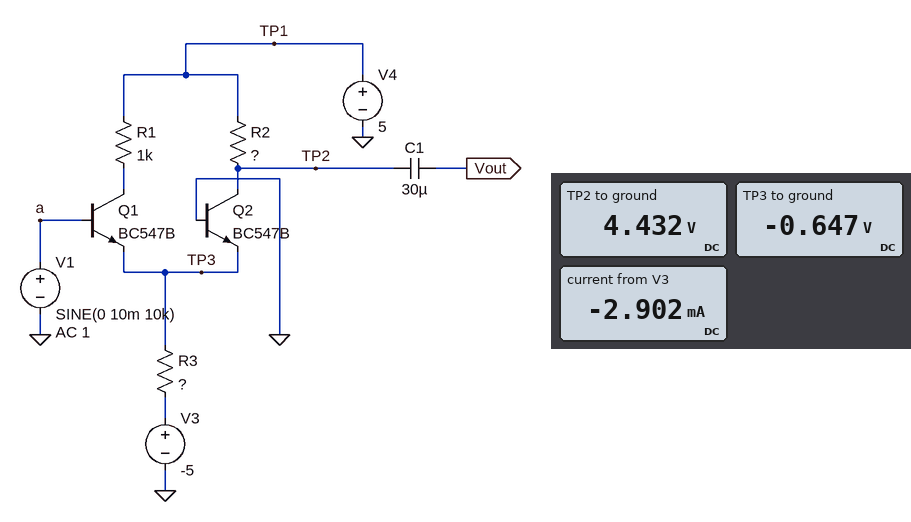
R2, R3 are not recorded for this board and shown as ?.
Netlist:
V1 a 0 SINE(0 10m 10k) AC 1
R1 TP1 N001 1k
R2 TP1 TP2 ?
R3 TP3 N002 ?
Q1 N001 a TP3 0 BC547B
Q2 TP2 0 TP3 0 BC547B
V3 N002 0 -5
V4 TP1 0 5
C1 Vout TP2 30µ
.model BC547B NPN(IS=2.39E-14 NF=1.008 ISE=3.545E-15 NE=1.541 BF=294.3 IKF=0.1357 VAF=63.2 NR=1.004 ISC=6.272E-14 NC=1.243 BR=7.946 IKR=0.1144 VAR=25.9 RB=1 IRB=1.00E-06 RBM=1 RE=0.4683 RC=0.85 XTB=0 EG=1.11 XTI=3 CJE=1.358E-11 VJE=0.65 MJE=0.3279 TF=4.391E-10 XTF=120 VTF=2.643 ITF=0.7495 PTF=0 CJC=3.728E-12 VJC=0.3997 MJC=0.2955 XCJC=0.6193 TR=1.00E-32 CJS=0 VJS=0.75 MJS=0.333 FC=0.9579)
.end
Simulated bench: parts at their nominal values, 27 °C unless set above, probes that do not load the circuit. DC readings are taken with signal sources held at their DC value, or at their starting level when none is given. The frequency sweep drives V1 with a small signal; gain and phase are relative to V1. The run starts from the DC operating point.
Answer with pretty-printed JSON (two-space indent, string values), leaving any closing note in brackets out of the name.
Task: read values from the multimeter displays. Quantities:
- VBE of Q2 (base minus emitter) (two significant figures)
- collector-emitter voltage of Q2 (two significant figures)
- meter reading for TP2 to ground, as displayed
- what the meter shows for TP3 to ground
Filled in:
{
  "VBE of Q2 (base minus emitter)": "650 mV",
  "collector-emitter voltage of Q2": "5.1 V",
  "meter reading for TP2 to ground, as displayed": "4.432 V",
  "what the meter shows for TP3 to ground": "-0.647 V"
}
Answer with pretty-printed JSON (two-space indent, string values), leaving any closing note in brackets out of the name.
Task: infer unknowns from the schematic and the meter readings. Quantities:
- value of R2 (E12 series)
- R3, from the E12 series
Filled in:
{
  "value of R2": "390 Ω",
  "R3, from the E12 series": "1.5 kΩ"
}
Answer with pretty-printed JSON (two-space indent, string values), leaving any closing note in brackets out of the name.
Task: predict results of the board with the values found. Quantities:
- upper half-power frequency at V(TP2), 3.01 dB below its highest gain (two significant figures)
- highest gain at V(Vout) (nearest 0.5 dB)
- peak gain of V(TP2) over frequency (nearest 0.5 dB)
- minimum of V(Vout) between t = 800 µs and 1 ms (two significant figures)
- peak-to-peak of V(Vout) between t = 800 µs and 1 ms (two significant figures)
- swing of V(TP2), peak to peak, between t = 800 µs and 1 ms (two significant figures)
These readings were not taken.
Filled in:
{
  "upper half-power frequency at V(TP2), 3.01 dB below its highest gain": "220 MHz",
  "highest gain at V(Vout)": "20.0 dB",
  "peak gain of V(TP2) over frequency": "20.0 dB",
  "minimum of V(Vout) between t = 800 µs and 1 ms": "-100 mV",
  "peak-to-peak of V(Vout) between t = 800 µs and 1 ms": "200 mV",
  "swing of V(TP2), peak to peak, between t = 800 µs and 1 ms": "200 mV"
}
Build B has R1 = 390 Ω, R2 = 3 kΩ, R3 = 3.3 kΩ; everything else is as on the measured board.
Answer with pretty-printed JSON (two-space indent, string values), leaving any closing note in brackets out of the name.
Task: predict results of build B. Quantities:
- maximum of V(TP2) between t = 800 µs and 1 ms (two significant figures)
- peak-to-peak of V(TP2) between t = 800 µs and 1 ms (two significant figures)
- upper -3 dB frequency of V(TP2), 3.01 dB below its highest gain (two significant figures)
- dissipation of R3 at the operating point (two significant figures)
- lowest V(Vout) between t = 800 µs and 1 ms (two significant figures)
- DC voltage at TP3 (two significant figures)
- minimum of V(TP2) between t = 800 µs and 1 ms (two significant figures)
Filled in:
{
  "maximum of V(TP2) between t = 800 µs and 1 ms": "3.4 V",
  "peak-to-peak of V(TP2) between t = 800 µs and 1 ms": "720 mV",
  "upper -3 dB frequency of V(TP2), 3.01 dB below its highest gain": "27 MHz",
  "dissipation of R3 at the operating point": "5.8 mW",
  "lowest V(Vout) between t = 800 µs and 1 ms": "-360 mV",
  "DC voltage at TP3": "-630 mV",
  "minimum of V(TP2) between t = 800 µs and 1 ms": "2.7 V"
}
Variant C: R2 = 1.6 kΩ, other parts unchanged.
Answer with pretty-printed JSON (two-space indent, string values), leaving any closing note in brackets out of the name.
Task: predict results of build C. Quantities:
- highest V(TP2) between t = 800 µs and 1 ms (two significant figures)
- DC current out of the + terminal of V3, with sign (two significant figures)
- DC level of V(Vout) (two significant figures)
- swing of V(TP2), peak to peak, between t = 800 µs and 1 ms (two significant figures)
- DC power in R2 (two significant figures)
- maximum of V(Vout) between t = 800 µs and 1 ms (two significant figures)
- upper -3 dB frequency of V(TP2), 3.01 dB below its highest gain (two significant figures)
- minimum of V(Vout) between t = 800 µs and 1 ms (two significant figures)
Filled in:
{
  "highest V(TP2) between t = 800 µs and 1 ms": "3.1 V",
  "DC current out of the + terminal of V3, with sign": "-2.9 mA",
  "DC level of V(Vout)": "2.7 V",
  "swing of V(TP2), peak to peak, between t = 800 µs and 1 ms": "820 mV",
  "DC power in R2": "3.3 mW",
  "maximum of V(Vout) between t = 800 µs and 1 ms": "410 mV",
  "upper -3 dB frequency of V(TP2), 3.01 dB below its highest gain": "49 MHz",
  "minimum of V(Vout) between t = 800 µs and 1 ms": "-410 mV"
}
